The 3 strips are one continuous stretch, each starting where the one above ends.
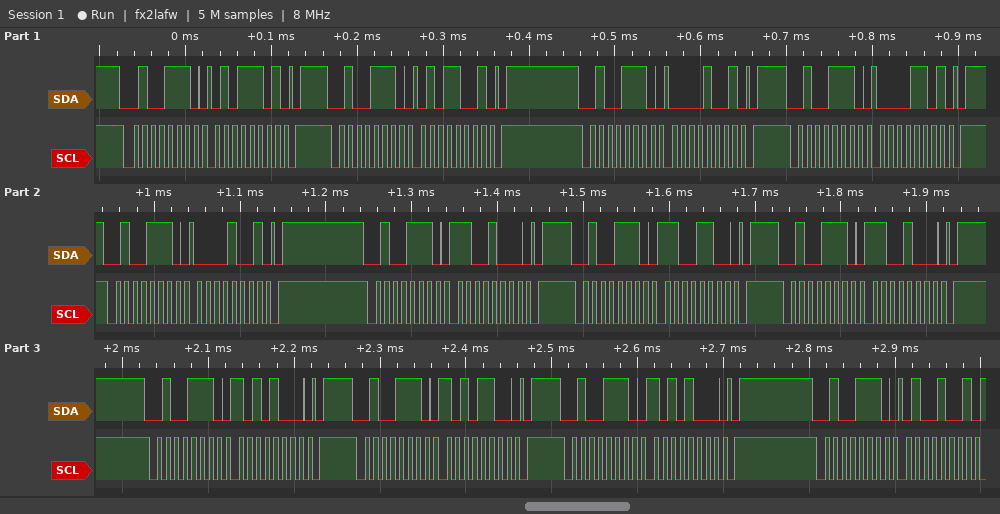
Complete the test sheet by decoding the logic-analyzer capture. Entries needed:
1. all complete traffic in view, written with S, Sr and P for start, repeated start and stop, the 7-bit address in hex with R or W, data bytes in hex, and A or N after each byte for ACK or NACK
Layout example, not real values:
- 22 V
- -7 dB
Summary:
- S 27W A 5D A P S 27W A 59 A P S 27W A 09 A P S 27W A 0D A P S 27W A 09 A P S 27W A C8 A P S 27W A CC A P S 27W A C8 A P S 27W A A8 A P S 27W A AC A P S 27W A A8 A P S 27W A 49 A
